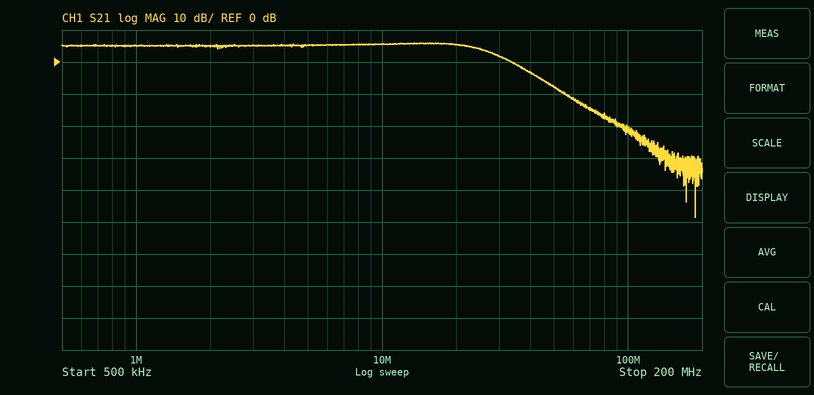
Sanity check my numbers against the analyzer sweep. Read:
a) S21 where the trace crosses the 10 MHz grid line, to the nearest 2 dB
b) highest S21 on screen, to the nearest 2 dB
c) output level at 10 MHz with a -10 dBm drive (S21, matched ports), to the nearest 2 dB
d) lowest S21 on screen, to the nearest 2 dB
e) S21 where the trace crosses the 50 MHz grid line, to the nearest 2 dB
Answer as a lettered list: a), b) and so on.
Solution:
a) 6 dB
b) 6 dB
c) -4 dBm
d) -48 dB
e) -8 dB
